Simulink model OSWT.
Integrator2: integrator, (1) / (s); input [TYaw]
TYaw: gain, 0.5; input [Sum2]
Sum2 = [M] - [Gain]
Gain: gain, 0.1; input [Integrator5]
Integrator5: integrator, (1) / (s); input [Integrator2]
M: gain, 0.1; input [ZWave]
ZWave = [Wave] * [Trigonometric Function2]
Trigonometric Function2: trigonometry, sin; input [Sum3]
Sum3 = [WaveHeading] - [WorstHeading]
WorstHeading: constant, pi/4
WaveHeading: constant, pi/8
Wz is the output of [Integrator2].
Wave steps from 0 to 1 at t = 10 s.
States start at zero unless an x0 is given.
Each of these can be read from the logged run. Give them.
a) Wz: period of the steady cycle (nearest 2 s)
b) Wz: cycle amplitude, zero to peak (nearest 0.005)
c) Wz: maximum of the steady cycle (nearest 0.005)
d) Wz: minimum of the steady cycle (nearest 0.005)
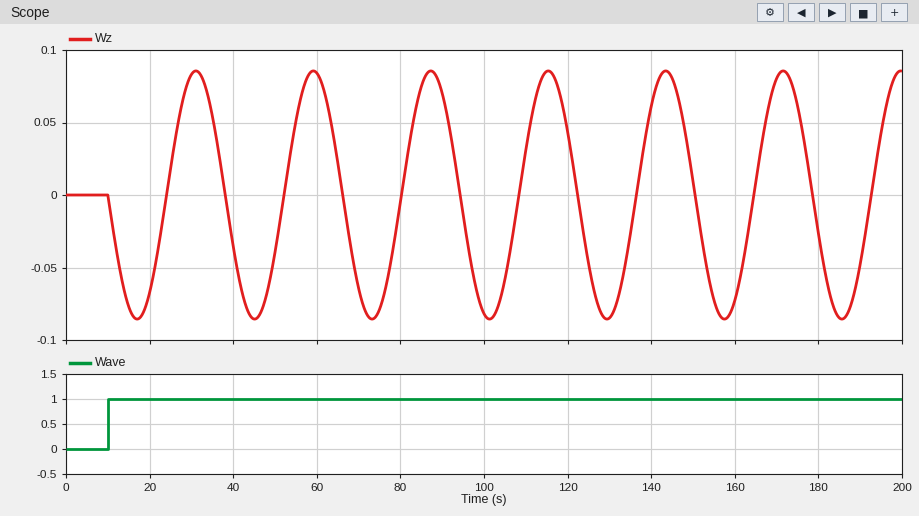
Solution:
28 s
0.085
0.085
-0.085
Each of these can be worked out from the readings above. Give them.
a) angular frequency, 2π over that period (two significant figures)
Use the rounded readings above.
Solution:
0.22 rad/s
